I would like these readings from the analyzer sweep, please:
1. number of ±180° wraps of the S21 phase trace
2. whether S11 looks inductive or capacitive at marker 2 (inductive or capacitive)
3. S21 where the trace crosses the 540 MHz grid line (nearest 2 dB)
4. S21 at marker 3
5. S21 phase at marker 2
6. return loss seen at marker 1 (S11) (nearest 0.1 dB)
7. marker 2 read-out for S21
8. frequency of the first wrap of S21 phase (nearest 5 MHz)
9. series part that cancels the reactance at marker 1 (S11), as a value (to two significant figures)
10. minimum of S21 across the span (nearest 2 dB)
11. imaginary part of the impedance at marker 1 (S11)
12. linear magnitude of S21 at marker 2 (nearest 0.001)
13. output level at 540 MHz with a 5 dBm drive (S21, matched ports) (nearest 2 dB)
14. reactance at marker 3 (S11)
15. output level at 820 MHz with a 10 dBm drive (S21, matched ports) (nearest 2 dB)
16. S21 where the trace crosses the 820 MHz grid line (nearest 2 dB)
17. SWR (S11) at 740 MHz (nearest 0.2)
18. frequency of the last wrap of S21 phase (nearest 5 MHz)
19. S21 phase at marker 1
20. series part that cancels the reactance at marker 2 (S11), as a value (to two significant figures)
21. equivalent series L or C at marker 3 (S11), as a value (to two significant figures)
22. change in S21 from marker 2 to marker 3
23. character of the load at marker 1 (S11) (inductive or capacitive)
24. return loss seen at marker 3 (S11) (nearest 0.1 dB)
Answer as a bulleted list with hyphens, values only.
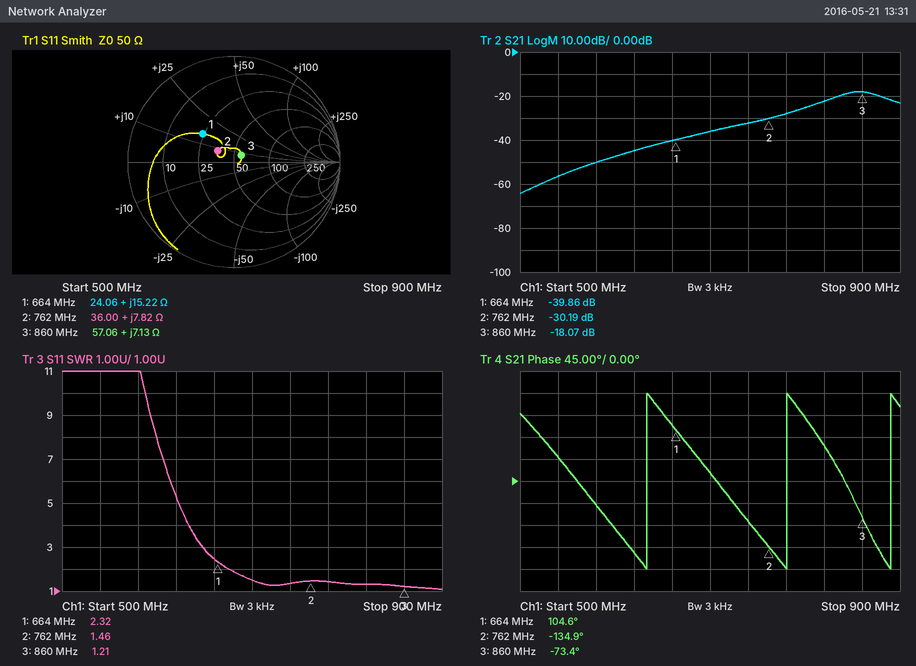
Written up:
- 3
- inductive
- -56 dB
- -18.07 dB
- -134.9°
- 8.0 dB
- -30.19 dB
- 635 MHz
- 16 pF
- -64 dB
- +15.22 Ω
- 0.031
- -52 dBm
- +7.13 Ω
- -12 dBm
- -22 dB
- 1.4
- 890 MHz
- 104.6°
- 27 pF
- 1.3 nH
- 12.12 dB
- inductive
- 20.6 dB
